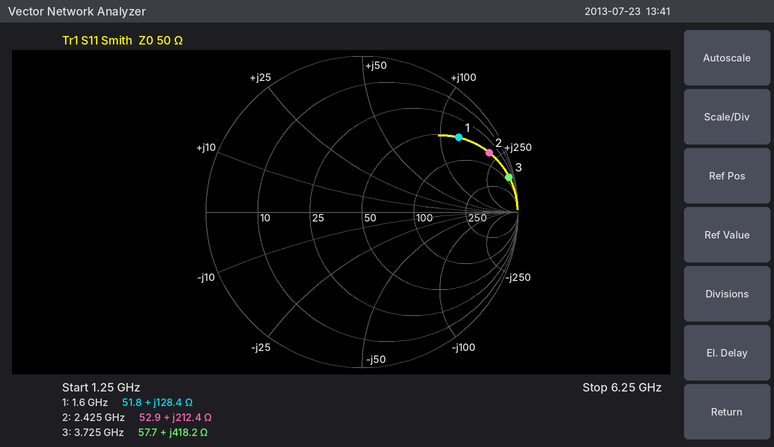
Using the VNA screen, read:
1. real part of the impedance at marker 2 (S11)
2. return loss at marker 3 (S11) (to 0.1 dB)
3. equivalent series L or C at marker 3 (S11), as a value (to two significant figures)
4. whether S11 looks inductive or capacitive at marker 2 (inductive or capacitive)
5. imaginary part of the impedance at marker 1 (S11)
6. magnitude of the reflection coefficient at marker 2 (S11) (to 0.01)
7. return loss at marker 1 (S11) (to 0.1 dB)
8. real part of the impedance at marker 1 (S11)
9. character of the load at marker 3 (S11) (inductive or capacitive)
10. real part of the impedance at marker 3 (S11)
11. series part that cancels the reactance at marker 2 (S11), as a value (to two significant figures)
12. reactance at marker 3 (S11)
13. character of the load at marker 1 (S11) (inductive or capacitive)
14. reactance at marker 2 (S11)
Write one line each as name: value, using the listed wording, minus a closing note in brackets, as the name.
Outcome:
real part of the impedance at marker 2: 52.9 Ω
return loss at marker 3 (S11): 0.3 dB
equivalent series L or C at marker 3 (S11), as a value: 18 nH
whether S11 looks inductive or capacitive at marker 2: inductive
imaginary part of the impedance at marker 1: +128.4 Ω
magnitude of the reflection coefficient at marker 2 (S11): 0.90
return loss at marker 1 (S11): 2.1 dB
real part of the impedance at marker 1: 51.8 Ω
character of the load at marker 3 (S11): inductive
real part of the impedance at marker 3: 57.7 Ω
series part that cancels the reactance at marker 2 (S11), as a value: 310 fF
reactance at marker 3: +418.2 Ω
character of the load at marker 1 (S11): inductive
reactance at marker 2: +212.4 Ω
